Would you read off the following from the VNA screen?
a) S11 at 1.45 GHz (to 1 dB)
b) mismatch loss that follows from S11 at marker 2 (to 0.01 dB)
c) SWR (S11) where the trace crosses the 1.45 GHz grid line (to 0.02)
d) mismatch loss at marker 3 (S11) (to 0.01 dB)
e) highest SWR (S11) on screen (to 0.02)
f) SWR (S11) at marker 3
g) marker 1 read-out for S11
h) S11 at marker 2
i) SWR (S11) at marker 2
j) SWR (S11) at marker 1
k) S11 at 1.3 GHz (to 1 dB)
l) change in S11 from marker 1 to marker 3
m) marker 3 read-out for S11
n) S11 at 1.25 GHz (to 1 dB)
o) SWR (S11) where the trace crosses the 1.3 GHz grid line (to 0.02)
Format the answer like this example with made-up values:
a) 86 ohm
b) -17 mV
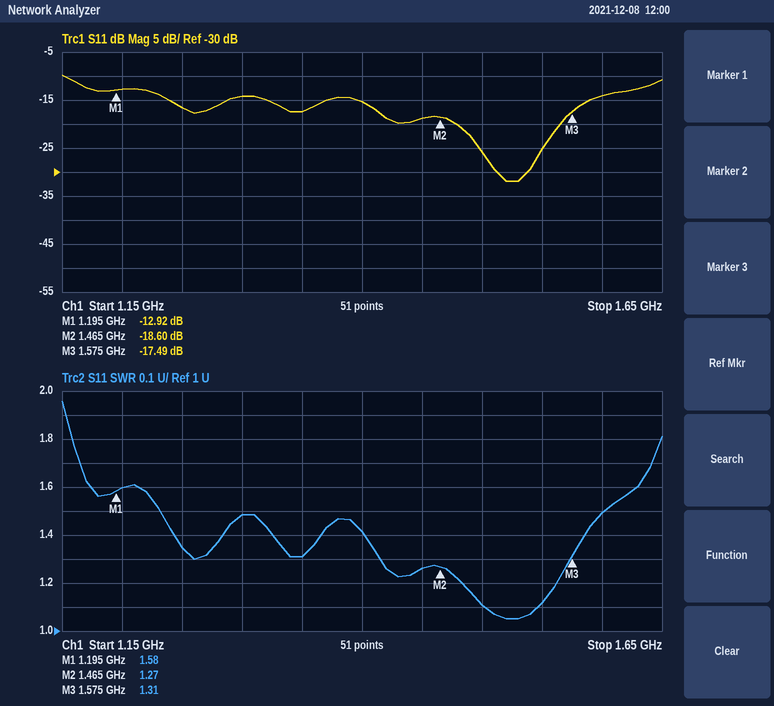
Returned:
a) -19 dB
b) 0.06 dB
c) 1.26
d) 0.08 dB
e) 1.96
f) 1.31
g) -12.92 dB
h) -18.60 dB
i) 1.27
j) 1.58
k) -14 dB
l) -4.57 dB
m) -17.49 dB
n) -17 dB
o) 1.48
